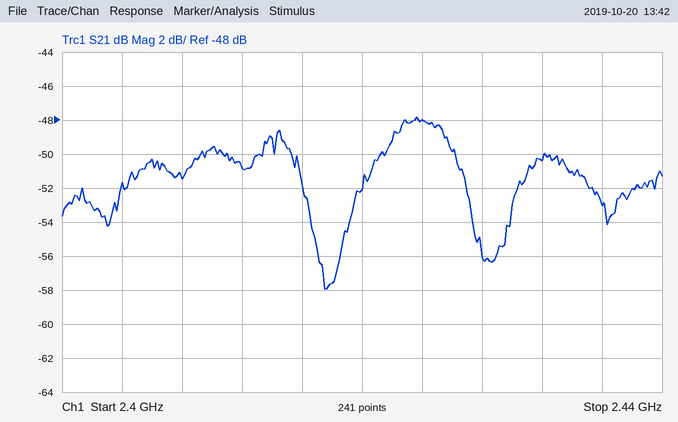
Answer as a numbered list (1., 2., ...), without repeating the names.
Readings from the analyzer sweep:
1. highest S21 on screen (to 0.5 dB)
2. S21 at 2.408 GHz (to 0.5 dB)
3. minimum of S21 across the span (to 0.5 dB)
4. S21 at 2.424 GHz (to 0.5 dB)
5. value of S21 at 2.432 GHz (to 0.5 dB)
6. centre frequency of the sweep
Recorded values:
1. -48.0 dB
2. -51.5 dB
3. -58.0 dB
4. -48.0 dB
5. -50.5 dB
6. 2.42 GHz
